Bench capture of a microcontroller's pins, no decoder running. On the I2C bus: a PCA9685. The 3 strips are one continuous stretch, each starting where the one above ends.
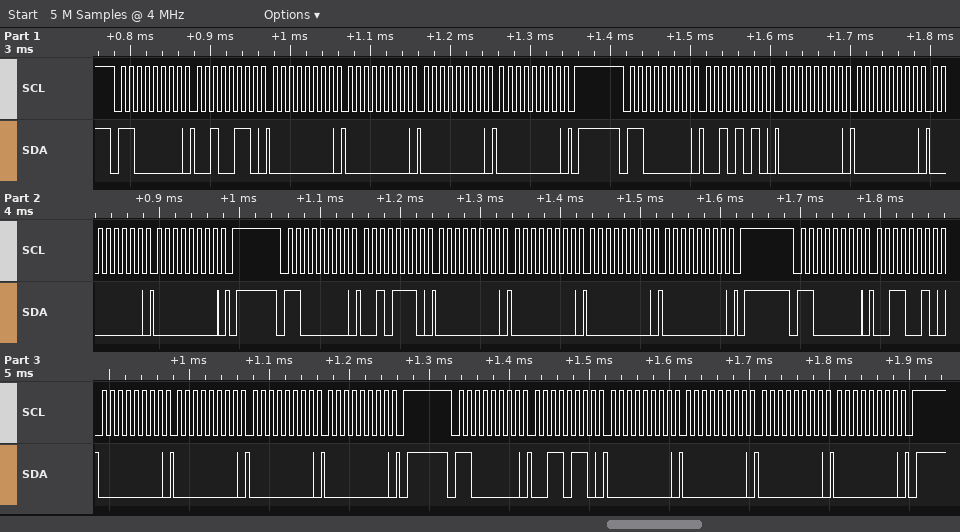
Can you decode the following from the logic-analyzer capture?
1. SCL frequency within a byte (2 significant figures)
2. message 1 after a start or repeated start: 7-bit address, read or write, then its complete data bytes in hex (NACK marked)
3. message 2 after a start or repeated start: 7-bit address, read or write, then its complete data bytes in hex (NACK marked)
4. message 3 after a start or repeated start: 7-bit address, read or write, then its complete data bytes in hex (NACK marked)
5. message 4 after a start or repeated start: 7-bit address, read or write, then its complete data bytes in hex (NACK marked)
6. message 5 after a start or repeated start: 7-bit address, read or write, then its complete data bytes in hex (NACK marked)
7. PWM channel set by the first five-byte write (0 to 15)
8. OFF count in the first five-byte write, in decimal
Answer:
100 kHz
0x60 write: 26 00 00 00 00
0x60 write: 2A 00 00 00 00
0x60 write: 2E 00 00 00 00
0x60 write: 32 00 00 00 00
0x60 write: 36 00 00 00 00
8
0
